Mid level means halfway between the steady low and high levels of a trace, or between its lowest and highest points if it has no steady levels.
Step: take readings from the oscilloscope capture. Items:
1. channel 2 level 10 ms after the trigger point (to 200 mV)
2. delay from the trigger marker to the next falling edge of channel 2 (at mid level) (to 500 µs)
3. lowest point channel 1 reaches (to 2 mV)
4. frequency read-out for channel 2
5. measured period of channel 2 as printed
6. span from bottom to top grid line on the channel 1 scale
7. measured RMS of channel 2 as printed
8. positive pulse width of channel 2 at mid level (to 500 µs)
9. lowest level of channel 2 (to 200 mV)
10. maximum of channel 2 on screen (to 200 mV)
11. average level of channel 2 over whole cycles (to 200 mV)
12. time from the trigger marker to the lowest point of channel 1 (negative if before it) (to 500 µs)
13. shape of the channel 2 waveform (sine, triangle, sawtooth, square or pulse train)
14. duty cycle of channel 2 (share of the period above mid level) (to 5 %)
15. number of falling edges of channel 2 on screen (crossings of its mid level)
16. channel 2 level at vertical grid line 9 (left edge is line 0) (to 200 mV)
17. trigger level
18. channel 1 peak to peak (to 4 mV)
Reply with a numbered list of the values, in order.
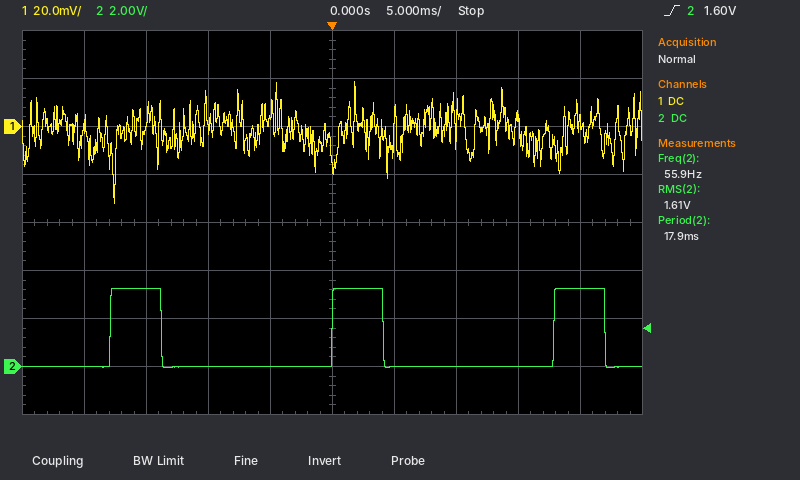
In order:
1. 0.0 V
2. 4.0 ms
3. -32 mV
4. 55.9 Hz
5. 17.9 ms
6. 160 mV
7. 1.61 V
8. 4.0 ms
9. 0.0 V
10. 3.2 V
11. 800 mV
12. -17.5 ms
13. pulse train
14. 25 %
15. 3
16. 3.2 V
17. 1.60 V
18. 52 mV
